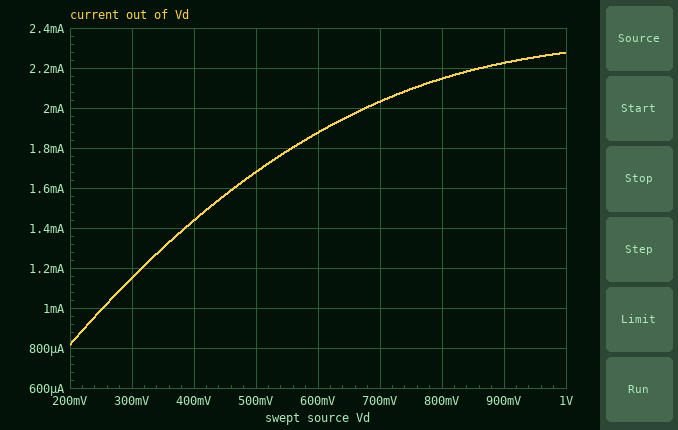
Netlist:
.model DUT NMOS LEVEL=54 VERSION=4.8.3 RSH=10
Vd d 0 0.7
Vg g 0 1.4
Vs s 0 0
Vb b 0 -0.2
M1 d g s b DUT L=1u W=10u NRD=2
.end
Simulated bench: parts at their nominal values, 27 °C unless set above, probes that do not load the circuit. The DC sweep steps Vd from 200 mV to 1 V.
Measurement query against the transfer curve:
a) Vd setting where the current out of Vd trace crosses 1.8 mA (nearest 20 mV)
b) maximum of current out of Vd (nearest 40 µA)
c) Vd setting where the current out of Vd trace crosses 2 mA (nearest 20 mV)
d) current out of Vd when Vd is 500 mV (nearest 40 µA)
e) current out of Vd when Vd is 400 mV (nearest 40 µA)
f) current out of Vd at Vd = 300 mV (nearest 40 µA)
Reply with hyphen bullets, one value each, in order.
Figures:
- 560 mV
- 2.28 mA
- 680 mV
- 1.68 mA
- 1.44 mA
- 1.16 mA
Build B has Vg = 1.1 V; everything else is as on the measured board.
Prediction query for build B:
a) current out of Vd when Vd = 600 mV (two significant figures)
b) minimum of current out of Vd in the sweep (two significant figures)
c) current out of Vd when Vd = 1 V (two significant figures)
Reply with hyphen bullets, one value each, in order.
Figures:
- 1.3 mA
- 640 µA
- 1.5 mA
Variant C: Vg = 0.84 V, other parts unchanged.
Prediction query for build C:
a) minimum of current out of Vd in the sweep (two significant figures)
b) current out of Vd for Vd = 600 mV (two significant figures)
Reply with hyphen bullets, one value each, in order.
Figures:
- 460 µA
- 800 µA
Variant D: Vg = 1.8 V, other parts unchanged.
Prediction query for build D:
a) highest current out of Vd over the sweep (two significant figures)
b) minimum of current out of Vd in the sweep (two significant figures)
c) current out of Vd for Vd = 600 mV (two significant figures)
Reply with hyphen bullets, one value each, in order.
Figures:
- 3.3 mA
- 1.0 mA
- 2.5 mA
